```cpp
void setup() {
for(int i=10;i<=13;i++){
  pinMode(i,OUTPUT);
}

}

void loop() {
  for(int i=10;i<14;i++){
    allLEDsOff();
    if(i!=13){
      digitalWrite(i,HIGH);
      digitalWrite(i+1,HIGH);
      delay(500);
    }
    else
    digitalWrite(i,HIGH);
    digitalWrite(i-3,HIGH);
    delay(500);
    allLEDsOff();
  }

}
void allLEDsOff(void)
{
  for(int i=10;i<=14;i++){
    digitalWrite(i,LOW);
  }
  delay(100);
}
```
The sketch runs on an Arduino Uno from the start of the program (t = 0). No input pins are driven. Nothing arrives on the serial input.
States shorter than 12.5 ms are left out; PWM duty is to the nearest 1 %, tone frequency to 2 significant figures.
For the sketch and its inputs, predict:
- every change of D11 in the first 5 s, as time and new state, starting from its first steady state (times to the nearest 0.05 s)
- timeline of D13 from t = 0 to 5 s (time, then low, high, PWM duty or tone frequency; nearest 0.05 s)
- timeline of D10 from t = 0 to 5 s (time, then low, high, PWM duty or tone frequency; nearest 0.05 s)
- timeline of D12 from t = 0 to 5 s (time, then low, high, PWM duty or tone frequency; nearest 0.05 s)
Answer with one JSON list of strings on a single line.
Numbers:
["0 s low; 0.1 s high; 1.1 s low; 1.3 s high; 2.3 s low; 4.4 s high", "0 s low; 2.5 s high; 3.5 s low; 3.7 s high; 4.2 s low", "0 s low; 0.1 s high; 1.1 s low; 3.7 s high; 4.2 s low; 4.4 s high", "0 s low; 1.3 s high; 2.3 s low; 2.5 s high; 3.5 s low"]
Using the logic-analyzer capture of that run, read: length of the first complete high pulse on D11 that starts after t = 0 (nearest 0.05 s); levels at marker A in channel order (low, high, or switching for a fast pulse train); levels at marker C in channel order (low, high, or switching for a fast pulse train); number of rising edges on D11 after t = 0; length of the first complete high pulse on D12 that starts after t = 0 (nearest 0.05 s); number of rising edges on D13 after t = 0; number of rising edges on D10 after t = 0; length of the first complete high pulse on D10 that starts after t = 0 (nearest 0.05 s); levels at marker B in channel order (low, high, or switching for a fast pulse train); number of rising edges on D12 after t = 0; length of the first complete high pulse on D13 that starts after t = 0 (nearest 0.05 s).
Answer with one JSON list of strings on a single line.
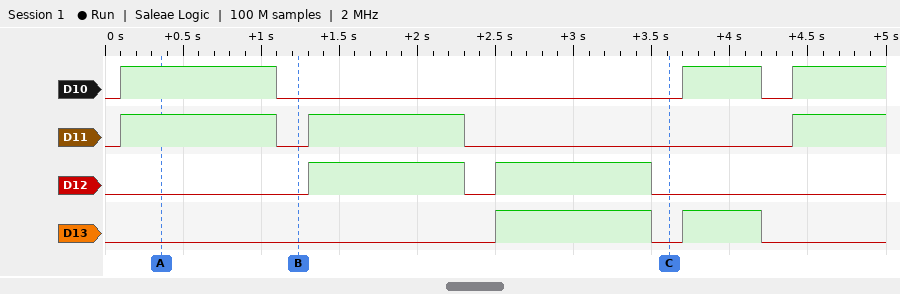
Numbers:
["1.00 s", "D10 high, D11 high, D12 low, D13 low", "D10 low, D11 low, D12 low, D13 low", "3", "1.00 s", "2", "3", "1.00 s", "D10 low, D11 low, D12 low, D13 low", "2", "1.00 s"]
